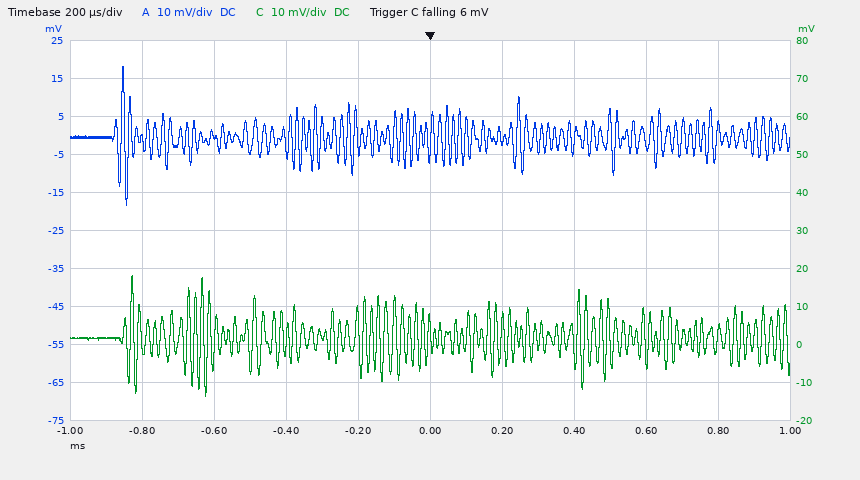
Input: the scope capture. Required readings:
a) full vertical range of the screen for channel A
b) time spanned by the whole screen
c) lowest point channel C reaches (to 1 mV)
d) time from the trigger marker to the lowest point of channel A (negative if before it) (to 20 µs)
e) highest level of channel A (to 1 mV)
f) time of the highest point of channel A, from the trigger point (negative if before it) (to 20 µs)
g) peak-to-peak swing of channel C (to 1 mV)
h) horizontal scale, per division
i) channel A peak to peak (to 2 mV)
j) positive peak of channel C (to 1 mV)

100 mV
2 ms
-14 mV
-840 µs
18 mV
-860 µs
32 mV
200 µs
36 mV
18 mV
